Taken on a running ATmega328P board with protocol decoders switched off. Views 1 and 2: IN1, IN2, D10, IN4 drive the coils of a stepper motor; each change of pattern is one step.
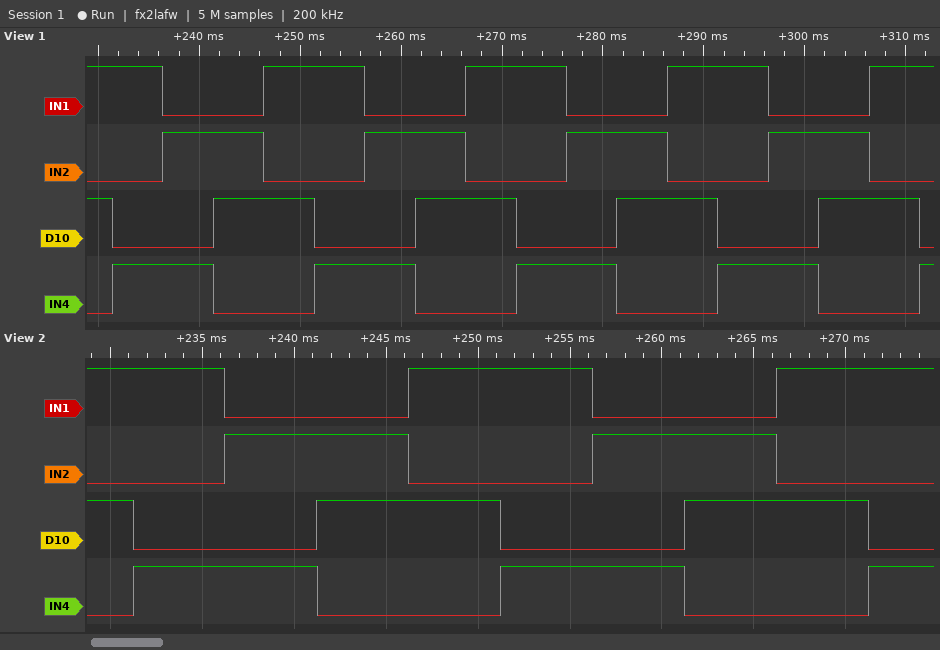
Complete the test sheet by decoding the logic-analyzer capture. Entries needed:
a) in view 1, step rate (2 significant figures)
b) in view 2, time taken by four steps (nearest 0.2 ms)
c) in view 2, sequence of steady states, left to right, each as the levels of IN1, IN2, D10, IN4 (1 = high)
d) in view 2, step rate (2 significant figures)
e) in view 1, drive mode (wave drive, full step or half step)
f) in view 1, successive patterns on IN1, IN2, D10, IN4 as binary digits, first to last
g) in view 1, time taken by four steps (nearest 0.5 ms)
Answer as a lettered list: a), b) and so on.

a) 200 steps/s
b) 20.0 ms
c) 1010 1001 0101 0110 1010 1001 0101 0110 1010 1001
d) 200 steps/s
e) full step
f) 1010 1001 0101 0110 1010 1001 0101 0110 1010 1001 0101 0110 1010 1001 0101 0110 1010 1001
g) 20.0 ms
